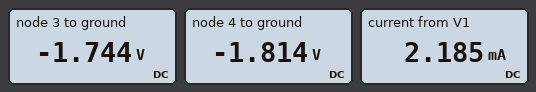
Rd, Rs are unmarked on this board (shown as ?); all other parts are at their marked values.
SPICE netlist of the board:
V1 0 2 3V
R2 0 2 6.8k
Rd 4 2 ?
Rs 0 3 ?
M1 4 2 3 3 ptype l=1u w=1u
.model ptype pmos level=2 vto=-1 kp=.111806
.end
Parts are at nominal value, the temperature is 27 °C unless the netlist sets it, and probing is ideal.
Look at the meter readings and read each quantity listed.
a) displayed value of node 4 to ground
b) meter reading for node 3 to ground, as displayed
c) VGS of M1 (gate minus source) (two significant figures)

-1.814 V
-1.744 V
-1.3 V
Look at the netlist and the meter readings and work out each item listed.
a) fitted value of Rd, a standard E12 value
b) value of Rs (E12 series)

680 Ω
1 kΩ
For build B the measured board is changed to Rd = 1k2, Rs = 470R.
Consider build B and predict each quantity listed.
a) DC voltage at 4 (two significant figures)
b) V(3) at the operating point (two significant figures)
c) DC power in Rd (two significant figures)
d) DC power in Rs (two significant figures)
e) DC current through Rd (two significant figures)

-850 mV
-840 mV
3.8 mW
1.5 mW
1.8 mA
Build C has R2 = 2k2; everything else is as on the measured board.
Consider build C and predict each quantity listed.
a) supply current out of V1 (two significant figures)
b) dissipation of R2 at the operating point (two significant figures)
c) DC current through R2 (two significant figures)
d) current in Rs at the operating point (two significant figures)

3.1 mA
4.1 mW
1.4 mA
1.7 mA
